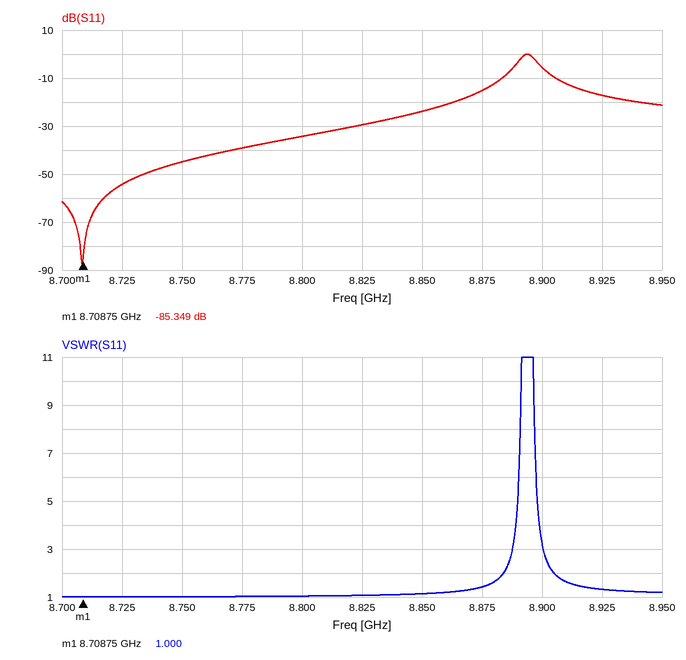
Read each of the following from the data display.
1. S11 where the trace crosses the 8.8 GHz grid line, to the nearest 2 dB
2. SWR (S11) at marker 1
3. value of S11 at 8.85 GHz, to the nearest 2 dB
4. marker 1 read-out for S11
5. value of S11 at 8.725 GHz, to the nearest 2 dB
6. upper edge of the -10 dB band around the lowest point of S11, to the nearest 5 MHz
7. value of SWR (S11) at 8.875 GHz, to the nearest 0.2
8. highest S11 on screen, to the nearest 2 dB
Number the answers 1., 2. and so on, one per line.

1. -34 dB
2. 1.000
3. -24 dB
4. -85.349 dB
5. -54 dB
6. 8.885 GHz
7. 1.4
8. 0 dB
